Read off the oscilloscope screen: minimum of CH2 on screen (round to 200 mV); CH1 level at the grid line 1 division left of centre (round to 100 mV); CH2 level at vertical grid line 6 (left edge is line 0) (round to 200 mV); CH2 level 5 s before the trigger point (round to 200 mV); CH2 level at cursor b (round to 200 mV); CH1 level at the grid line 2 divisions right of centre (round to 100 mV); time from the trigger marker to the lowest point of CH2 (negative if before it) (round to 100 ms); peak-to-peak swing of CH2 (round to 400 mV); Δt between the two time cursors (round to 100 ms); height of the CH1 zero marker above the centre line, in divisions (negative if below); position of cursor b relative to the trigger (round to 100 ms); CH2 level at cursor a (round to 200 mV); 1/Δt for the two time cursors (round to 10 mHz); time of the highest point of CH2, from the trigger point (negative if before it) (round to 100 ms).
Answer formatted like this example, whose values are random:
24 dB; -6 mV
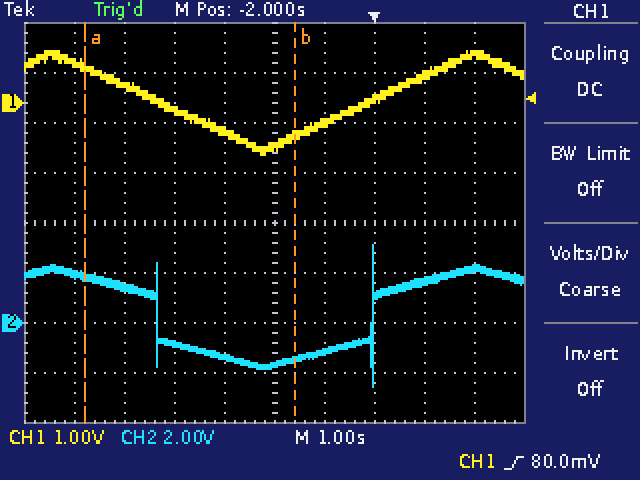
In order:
-2.6 V; -600 mV; -1.2 V; 1.4 V; -1.4 V; 100 mV; 0.0 s; 5.6 V; 4.2 s; +2.4 div; -1.6 s; 1.8 V; 240 mHz; 0.0 s
